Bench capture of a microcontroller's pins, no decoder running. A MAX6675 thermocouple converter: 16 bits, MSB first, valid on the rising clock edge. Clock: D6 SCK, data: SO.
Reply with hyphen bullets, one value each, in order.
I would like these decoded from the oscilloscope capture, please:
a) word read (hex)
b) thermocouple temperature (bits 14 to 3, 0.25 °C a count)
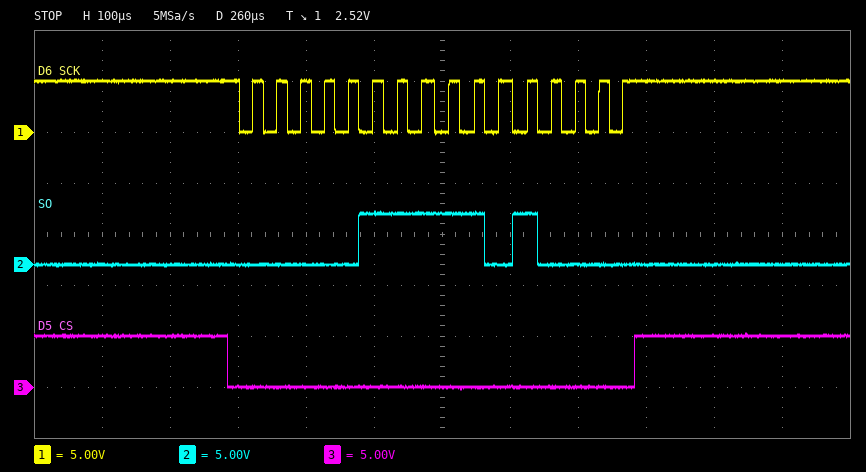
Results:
- 0x07D0
- 62.50 °C
